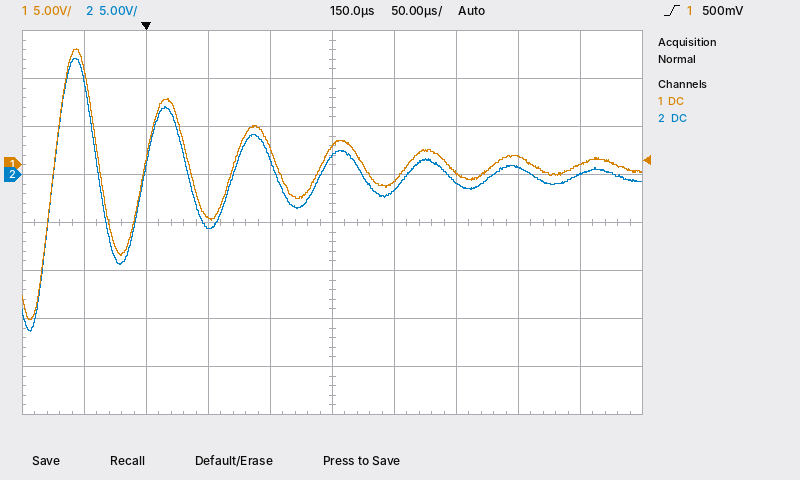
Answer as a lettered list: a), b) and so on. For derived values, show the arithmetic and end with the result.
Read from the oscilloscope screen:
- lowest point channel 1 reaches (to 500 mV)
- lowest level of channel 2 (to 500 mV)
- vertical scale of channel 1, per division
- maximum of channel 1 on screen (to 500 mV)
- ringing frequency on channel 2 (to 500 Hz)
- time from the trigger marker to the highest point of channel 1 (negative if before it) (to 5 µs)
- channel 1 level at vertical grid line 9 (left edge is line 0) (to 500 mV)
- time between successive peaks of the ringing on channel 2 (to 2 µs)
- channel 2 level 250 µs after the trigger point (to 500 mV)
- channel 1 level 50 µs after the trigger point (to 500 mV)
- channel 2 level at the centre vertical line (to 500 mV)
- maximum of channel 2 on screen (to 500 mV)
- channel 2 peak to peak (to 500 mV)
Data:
a) -16.0 V
b) -16.5 V
c) 5 V
d) 12.0 V
e) 1 / 70 µs ≈ 14.3 kHz, so 14.5 kHz to the nearest 500 Hz
f) -55 µs
g) 0.0 V
h) 70 µs
i) -1.0 V
j) -5.5 V
k) 2.0 V
l) 12.0 V
m) 12.0 V − (-16.5 V) = 28.5 V
